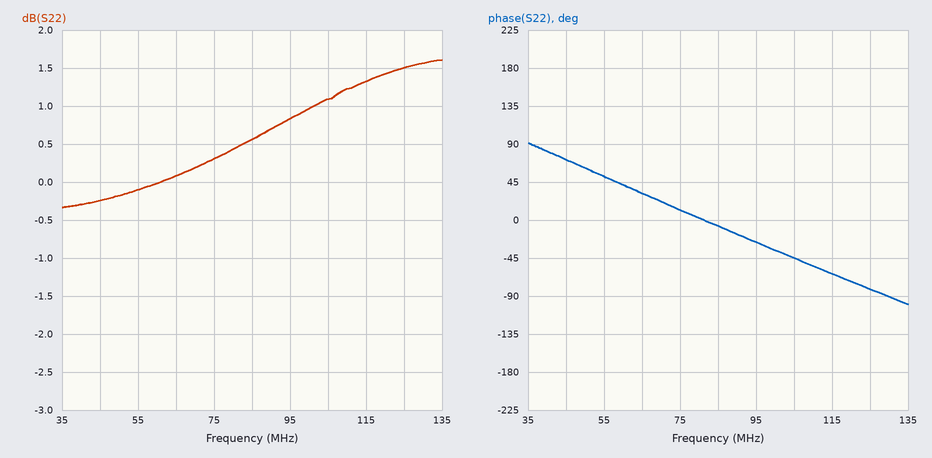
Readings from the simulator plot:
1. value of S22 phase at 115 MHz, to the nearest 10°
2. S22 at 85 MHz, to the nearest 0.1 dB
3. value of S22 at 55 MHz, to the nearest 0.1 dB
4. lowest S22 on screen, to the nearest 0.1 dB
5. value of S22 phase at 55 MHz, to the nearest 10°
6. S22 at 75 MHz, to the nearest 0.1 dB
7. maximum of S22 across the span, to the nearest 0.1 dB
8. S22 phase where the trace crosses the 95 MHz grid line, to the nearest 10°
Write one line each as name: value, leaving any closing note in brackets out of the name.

value of S22 phase at 115 MHz, to the nearest 10°: -60°
S22 at 85 MHz, to the nearest 0.1 dB: 0.6 dB
value of S22 at 55 MHz, to the nearest 0.1 dB: -0.1 dB
lowest S22 on screen, to the nearest 0.1 dB: -0.3 dB
value of S22 phase at 55 MHz, to the nearest 10°: 50°
S22 at 75 MHz, to the nearest 0.1 dB: 0.3 dB
maximum of S22 across the span, to the nearest 0.1 dB: 1.6 dB
S22 phase where the trace crosses the 95 MHz grid line, to the nearest 10°: -30°
